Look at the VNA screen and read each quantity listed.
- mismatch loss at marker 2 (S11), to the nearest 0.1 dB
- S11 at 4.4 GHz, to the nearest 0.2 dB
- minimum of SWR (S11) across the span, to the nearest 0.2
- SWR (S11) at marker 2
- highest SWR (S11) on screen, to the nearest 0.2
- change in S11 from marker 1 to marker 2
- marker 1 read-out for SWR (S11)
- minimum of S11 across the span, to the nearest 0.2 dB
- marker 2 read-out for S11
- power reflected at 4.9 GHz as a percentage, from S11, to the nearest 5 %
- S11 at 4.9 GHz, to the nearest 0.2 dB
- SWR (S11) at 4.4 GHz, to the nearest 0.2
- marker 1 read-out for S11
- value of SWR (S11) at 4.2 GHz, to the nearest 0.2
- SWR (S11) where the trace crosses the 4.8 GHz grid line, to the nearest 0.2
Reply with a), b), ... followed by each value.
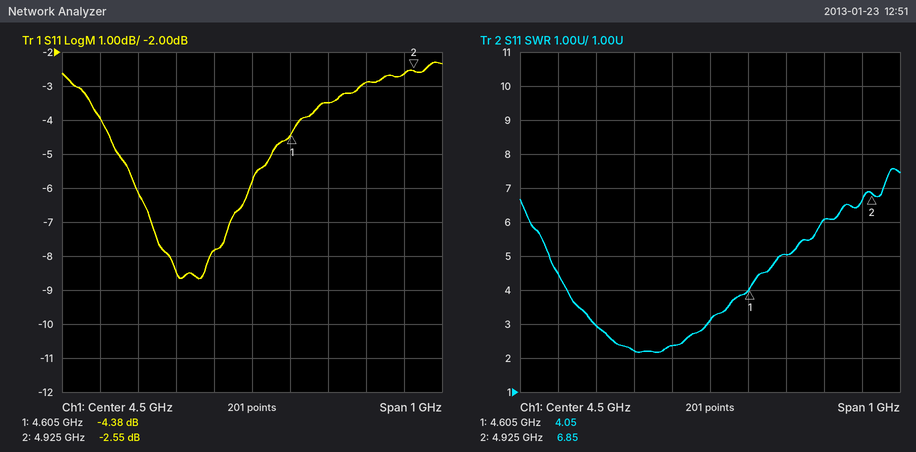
a) 3.5 dB
b) -7.8 dB
c) 2.2
d) 6.85
e) 7.6
f) 1.83 dB
g) 4.05
h) -8.6 dB
i) -2.55 dB
j) 55 %
k) -2.6 dB
l) 2.4
m) -4.38 dB
n) 3.0
o) 6.0
